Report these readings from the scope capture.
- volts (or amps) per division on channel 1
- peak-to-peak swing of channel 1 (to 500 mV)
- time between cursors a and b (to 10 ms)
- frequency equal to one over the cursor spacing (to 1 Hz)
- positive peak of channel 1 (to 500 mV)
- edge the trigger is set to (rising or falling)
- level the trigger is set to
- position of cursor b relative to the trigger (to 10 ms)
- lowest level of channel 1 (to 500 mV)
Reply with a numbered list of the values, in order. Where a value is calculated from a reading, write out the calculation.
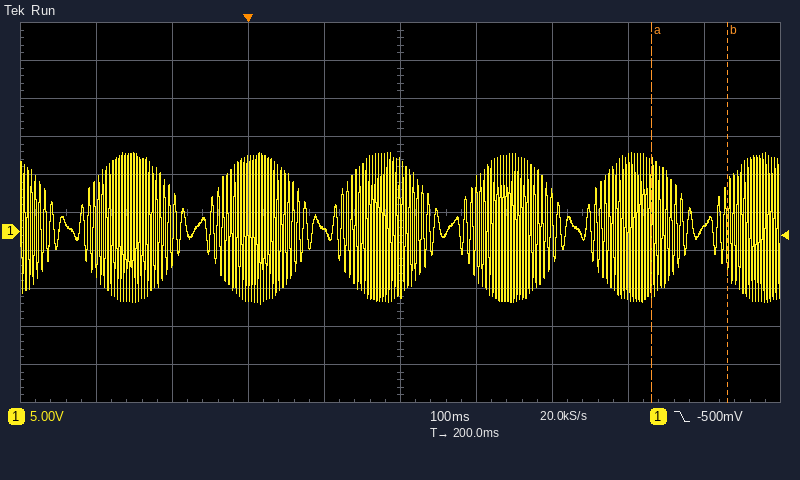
1. 5 V
2. 10.5 V − (-9.5 V) = 20.0 V
3. 100 ms
4. 1 / 100 ms ≈ 10 Hz
5. 10.5 V
6. falling
7. -500 mV
8. +630 ms
9. -9.5 V
